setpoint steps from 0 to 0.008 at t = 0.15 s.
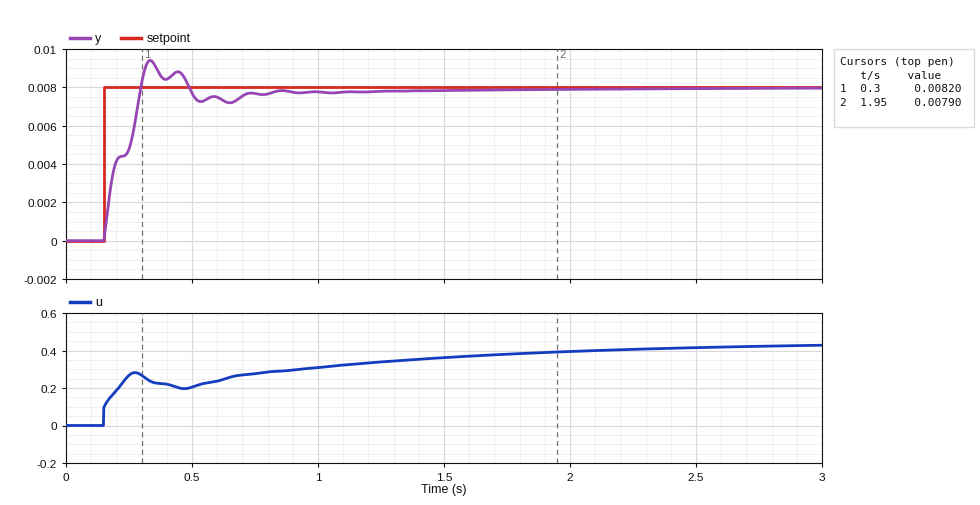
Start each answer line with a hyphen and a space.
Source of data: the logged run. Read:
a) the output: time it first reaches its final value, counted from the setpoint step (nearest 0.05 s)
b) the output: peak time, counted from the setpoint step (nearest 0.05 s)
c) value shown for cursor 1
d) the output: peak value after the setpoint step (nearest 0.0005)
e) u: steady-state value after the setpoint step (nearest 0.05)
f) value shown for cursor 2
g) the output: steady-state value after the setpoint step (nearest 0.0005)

- 0.15 s
- 0.20 s
- 0.00820
- 0.0095
- 0.45
- 0.00790
- 0.0080
